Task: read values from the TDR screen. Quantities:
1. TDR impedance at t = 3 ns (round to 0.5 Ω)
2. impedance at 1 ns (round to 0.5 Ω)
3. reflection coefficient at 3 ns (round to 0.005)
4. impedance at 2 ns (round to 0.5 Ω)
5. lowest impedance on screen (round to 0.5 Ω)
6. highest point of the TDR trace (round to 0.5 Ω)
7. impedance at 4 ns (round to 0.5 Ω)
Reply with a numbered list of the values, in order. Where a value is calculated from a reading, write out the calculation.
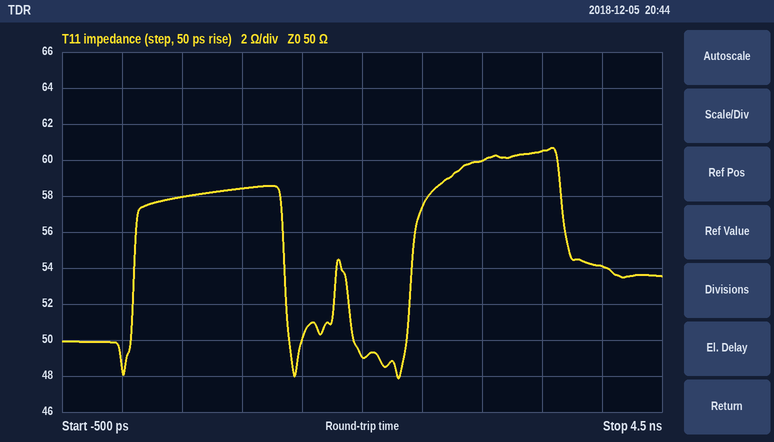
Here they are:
1. 60.0 Ω
2. 58.5 Ω
3. (60 − 50)/(60 + 50) ≈ +0.0909, so +0.090 to the nearest 0.005
4. 49.0 Ω
5. 48.0 Ω
6. 60.5 Ω
7. 54.0 Ω
